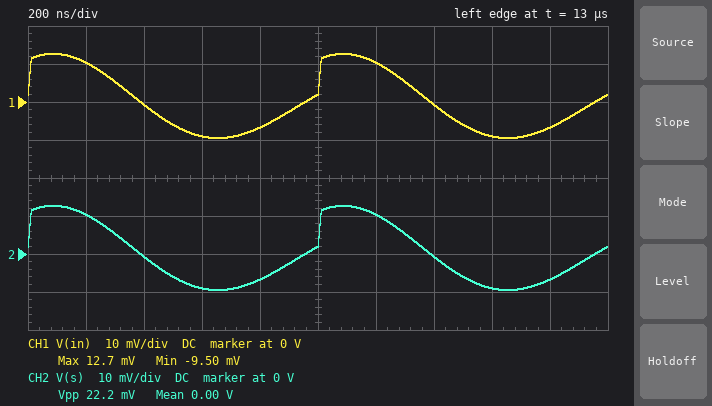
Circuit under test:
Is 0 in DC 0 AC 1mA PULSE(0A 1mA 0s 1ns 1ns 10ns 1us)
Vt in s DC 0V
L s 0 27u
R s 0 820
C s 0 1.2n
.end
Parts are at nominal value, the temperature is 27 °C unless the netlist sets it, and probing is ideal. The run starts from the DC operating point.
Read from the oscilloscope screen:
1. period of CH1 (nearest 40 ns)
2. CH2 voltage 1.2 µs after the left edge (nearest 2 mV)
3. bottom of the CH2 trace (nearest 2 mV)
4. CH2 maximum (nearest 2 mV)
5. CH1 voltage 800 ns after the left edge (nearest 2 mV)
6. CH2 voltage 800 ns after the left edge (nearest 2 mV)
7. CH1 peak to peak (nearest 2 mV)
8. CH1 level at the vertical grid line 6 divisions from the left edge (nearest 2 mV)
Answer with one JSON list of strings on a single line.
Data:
["1.00 µs", "10 mV", "-10 mV", "12 mV", "-6 mV", "-6 mV", "22 mV", "10 mV"]
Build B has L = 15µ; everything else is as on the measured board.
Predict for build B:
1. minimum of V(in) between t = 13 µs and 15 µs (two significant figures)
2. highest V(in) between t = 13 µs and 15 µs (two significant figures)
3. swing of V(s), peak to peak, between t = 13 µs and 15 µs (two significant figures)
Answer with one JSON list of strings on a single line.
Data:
["-8.3 mV", "7.2 mV", "16 mV"]
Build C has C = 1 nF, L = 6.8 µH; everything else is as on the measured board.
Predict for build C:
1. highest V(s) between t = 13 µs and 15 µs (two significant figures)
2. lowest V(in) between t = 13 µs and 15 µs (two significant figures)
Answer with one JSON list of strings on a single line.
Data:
["19 mV", "-16 mV"]
